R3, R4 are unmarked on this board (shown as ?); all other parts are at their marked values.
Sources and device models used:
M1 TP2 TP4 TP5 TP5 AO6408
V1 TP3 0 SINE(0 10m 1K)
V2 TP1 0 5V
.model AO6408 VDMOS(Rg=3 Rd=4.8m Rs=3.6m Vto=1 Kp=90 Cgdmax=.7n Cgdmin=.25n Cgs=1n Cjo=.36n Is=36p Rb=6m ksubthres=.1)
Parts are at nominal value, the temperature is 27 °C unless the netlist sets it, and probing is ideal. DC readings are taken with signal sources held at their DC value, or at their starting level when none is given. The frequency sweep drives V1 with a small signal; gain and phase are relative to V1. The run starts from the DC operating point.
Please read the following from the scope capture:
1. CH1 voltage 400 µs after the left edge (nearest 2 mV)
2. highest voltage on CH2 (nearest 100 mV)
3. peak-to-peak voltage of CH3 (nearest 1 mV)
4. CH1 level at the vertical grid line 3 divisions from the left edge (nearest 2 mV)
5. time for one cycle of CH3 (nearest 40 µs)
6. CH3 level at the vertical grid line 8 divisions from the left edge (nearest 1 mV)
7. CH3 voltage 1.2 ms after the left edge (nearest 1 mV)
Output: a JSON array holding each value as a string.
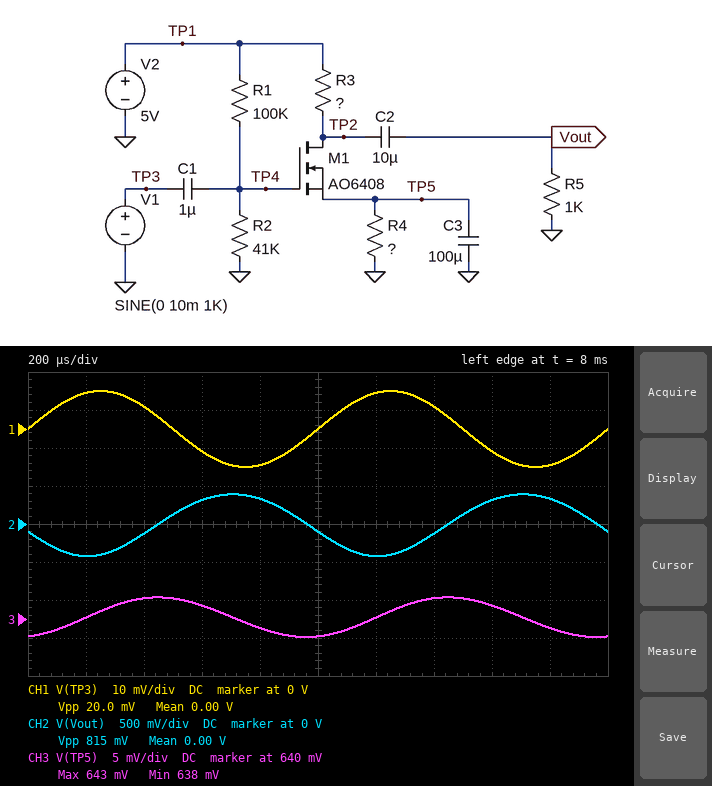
["6 mV", "400 mV", "5 mV", "-6 mV", "1.00 ms", "642 mV", "640 mV"]
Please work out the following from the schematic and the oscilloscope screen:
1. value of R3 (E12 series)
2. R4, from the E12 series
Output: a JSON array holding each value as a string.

["330 Ω", "68 Ω"]
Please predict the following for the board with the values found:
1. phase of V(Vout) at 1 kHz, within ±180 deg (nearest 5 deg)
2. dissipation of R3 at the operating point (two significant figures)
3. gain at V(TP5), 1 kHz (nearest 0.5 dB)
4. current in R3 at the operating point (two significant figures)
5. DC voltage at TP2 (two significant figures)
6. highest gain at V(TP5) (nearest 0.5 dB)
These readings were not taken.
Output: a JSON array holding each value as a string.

["-165 deg", "29 mW", "-11.5 dB", "9.4 mA", "1.9 V", "-1.0 dB"]
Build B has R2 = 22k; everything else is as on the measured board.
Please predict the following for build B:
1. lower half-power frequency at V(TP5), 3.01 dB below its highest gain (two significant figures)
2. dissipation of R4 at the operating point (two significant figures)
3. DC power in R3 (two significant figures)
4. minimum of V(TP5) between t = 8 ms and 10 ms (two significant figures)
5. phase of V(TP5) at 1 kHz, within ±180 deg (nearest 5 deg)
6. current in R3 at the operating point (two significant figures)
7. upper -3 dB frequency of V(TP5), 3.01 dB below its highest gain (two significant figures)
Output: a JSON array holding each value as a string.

["7.5 Hz", "380 µW", "1.8 mW", "160 mV", "-85 deg", "2.4 mA", "110 Hz"]
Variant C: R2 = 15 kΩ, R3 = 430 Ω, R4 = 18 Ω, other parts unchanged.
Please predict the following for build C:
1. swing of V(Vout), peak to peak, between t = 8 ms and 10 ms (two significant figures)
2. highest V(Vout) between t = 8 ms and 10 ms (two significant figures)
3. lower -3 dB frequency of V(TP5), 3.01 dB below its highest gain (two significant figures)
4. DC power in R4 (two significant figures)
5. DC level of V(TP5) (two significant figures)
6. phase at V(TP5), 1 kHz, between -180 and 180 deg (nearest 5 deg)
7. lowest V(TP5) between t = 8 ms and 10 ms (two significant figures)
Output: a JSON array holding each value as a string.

["43 mV", "20 mV", "10 Hz", "2.4 µW", "6.6 mV", "-85 deg", "6.5 mV"]
